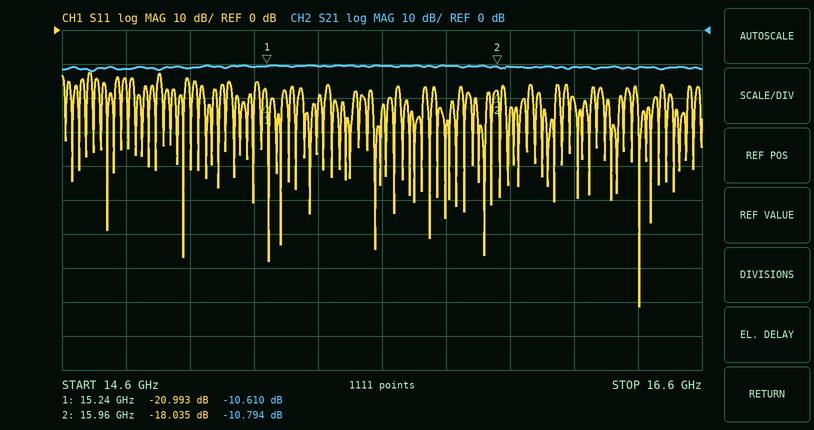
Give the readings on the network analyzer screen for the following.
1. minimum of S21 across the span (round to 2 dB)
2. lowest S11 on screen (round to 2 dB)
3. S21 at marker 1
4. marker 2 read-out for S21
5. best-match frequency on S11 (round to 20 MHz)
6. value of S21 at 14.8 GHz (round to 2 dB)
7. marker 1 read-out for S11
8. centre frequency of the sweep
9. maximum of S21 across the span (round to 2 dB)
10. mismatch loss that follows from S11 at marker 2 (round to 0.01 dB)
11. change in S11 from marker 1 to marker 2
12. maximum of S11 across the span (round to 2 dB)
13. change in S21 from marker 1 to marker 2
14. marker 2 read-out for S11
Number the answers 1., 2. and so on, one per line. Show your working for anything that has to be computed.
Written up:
1. -12 dB
2. -82 dB
3. -10.610 dB
4. -10.794 dB
5. 16.40 GHz
6. -12 dB
7. -20.993 dB
8. 15.6 GHz
9. -10 dB
10. −10 log10(1 − 10^(-18.035/10)) ≈ 0.07 dB
11. -18.035 − (-20.993) = 2.958 dB
12. -12 dB
13. -10.794 − (-10.61) = -0.184 dB
14. -18.035 dB
